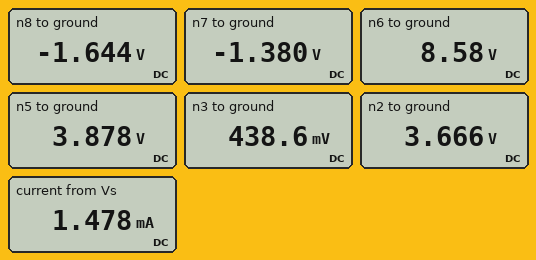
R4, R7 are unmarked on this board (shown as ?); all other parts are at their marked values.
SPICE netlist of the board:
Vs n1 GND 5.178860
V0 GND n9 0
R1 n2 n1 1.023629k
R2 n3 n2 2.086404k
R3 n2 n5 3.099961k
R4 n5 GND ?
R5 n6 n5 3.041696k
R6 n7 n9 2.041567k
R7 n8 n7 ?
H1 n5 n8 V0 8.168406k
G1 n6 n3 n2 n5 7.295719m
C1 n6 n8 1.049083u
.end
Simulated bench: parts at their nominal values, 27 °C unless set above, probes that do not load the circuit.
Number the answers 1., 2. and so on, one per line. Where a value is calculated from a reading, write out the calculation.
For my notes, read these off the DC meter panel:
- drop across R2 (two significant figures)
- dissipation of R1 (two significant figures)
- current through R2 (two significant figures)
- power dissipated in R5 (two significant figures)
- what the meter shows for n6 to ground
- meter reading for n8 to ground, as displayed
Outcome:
1. 3.666 V - 438.6 mV = 3.2 V
2. (5.179 V - 3.666 V)^2 / 1.024 kΩ = 2.2 mW
3. (3.666 V - 438.6 mV) / 2.086 kΩ = 1.5 mA
4. (8.58 V - 3.878 V)^2 / 3.042 kΩ = 7.3 mW
5. 8.58 V
6. -1.644 V
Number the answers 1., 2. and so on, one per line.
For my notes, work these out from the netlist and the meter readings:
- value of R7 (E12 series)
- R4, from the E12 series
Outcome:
1. 390 Ω
2. 1.8 kΩ
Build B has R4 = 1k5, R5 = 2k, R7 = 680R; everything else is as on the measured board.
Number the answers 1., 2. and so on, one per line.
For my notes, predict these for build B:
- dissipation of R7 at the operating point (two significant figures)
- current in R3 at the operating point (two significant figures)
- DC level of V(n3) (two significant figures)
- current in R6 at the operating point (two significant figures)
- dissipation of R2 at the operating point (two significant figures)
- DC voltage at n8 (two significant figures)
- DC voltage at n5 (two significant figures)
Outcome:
1. 300 µW
2. 81 µA
3. -450 mV
4. 670 µA
5. 7.0 mW
6. -1.8 V
7. 3.6 V
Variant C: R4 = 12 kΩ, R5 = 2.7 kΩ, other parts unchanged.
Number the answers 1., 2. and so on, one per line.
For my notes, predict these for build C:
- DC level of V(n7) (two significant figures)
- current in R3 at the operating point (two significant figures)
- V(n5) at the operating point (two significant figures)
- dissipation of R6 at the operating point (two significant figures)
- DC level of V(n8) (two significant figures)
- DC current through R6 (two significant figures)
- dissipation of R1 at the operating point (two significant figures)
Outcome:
1. -2.0 V
2. 24 µA
3. 5.6 V
4. 2.0 mW
5. -2.4 V
6. 980 µA
7. 270 µW
